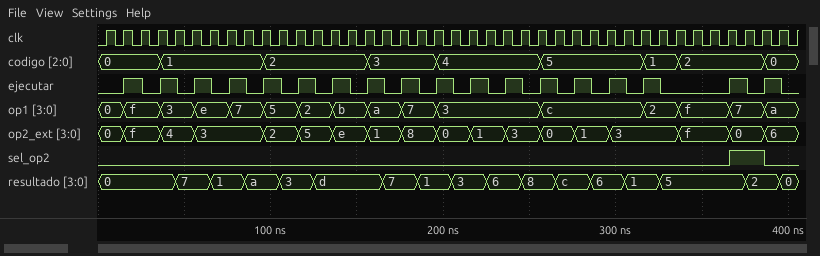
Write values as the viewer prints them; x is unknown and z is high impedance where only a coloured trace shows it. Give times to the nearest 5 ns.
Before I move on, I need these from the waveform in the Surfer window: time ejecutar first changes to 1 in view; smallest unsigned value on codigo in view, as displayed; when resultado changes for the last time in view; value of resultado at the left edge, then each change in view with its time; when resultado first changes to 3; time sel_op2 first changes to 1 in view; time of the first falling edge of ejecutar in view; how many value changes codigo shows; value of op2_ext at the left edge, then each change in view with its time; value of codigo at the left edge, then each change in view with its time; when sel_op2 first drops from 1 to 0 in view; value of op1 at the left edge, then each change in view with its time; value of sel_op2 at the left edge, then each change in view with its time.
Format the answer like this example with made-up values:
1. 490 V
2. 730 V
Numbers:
1. 15 ns
2. 0
3. 395 ns
4. 0, 7 at 45 ns, 1 at 65 ns, a at 85 ns, 3 at 105 ns, d at 125 ns, 7 at 165 ns, 1 at 185 ns, 3 at 205 ns, 6 at 225 ns, 8 at 245 ns, c at 265 ns, 6 at 285 ns, 1 at 305 ns, 5 at 325 ns, 2 at 375 ns, 0 at 395 ns
5. 105 ns
6. 365 ns
7. 25 ns
8. 8
9. 0, f at 15 ns, 4 at 35 ns, 3 at 55 ns, 2 at 95 ns, 5 at 115 ns, e at 135 ns, 1 at 155 ns, 8 at 175 ns, 0 at 195 ns, 1 at 215 ns, 3 at 235 ns, 0 at 255 ns, 1 at 275 ns, 3 at 295 ns, f at 335 ns, 0 at 365 ns, 6 at 385 ns
10. 0, 1 at 35 ns, 2 at 95 ns, 3 at 155 ns, 4 at 195 ns, 5 at 255 ns, 1 at 315 ns, 2 at 335 ns, 0 at 385 ns
11. 385 ns
12. 0, f at 15 ns, 3 at 35 ns, e at 55 ns, 7 at 75 ns, 5 at 95 ns, 2 at 115 ns, b at 135 ns, a at 155 ns, 7 at 175 ns, 3 at 195 ns, c at 255 ns, 2 at 315 ns, f at 335 ns, 7 at 365 ns, a at 385 ns
13. 0, 1 at 365 ns, 0 at 385 ns
